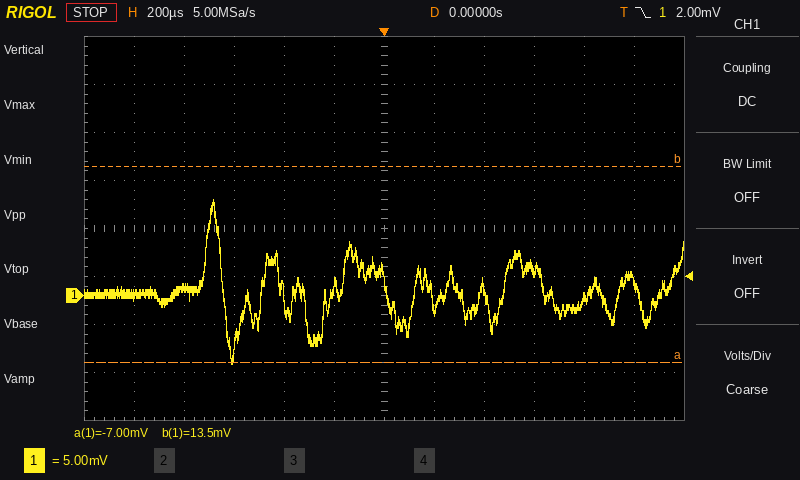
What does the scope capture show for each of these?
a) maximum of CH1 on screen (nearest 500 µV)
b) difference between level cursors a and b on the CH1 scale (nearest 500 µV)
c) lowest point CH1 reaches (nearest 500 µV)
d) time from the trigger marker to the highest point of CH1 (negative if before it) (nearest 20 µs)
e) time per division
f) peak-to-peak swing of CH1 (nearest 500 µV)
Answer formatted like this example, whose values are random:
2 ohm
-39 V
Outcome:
10.0 mV
20.5 mV
-7.0 mV
-680 µs
200 µs
17.0 mV
